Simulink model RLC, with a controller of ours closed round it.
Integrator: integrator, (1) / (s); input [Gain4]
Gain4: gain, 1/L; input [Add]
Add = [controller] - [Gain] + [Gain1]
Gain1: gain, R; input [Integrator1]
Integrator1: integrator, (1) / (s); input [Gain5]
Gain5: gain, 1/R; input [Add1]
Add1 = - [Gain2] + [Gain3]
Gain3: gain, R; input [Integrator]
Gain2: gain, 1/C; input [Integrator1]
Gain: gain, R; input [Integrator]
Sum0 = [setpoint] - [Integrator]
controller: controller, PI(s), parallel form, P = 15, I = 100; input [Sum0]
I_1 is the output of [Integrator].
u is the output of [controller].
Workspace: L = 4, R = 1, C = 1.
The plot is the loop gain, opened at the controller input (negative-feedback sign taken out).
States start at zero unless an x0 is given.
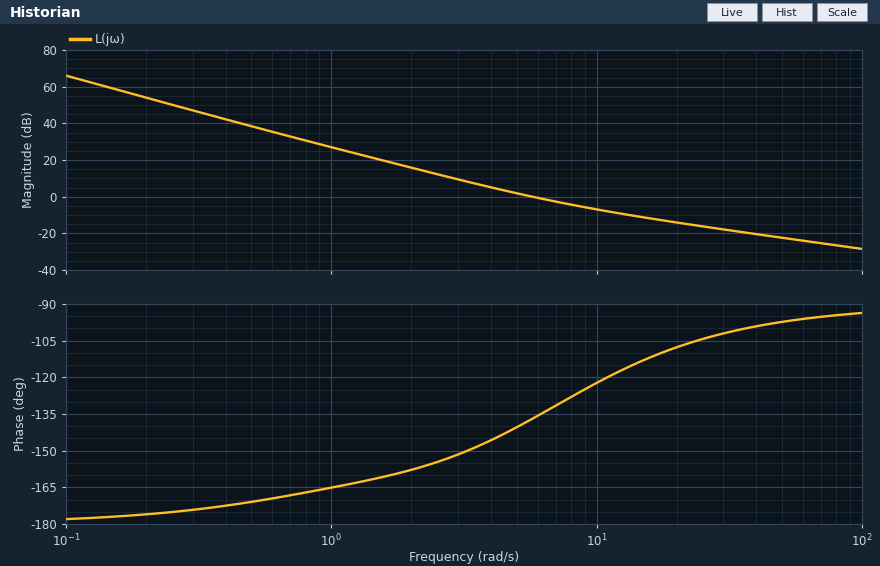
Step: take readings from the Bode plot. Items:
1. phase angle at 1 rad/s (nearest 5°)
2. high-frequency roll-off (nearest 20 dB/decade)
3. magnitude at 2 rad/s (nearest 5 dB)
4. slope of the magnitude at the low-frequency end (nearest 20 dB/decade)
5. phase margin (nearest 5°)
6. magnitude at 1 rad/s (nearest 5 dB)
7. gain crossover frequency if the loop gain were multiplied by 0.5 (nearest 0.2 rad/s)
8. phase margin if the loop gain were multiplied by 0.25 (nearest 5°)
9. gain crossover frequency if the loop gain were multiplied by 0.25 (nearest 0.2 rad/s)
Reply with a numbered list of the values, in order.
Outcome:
1. -165°
2. -20 dB/decade
3. 15 dB
4. -40 dB/decade
5. 45°
6. 25 dB
7. 3.8 rad/s
8. 25°
9. 2.6 rad/s
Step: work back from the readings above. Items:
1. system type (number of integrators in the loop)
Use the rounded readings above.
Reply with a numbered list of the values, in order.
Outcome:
1. 2
